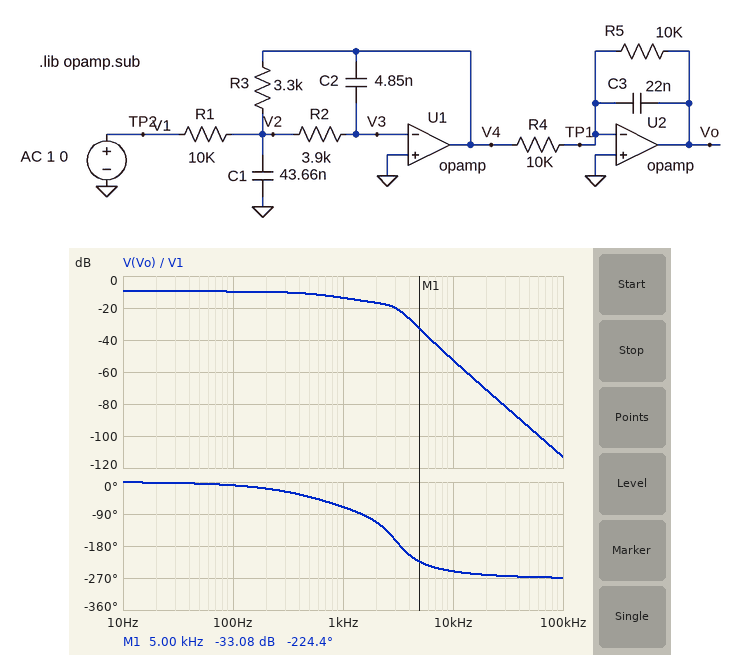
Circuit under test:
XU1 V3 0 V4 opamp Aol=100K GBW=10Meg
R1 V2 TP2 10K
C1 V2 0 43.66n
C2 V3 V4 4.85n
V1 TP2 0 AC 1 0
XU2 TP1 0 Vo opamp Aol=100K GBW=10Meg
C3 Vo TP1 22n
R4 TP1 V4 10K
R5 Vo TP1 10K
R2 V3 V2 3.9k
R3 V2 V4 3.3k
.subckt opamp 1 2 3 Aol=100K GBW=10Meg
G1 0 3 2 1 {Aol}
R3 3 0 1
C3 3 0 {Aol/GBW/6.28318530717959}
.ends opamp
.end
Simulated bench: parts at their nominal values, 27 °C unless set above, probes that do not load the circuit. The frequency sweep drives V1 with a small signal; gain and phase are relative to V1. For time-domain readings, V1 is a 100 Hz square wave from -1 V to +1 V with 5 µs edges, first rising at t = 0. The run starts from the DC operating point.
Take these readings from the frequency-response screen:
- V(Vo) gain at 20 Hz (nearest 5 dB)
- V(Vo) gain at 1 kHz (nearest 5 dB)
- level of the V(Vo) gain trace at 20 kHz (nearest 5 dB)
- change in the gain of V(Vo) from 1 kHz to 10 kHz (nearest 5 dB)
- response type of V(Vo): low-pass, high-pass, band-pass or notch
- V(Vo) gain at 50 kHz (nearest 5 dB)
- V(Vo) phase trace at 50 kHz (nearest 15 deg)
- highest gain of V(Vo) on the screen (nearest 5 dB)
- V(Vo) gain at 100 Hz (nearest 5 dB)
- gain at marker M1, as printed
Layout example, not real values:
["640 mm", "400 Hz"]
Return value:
["-10 dB", "-15 dB", "-70 dB", "-40 dB", "low-pass", "-95 dB", "-270 deg", "-10 dB", "-10 dB", "-33.08 dB"]
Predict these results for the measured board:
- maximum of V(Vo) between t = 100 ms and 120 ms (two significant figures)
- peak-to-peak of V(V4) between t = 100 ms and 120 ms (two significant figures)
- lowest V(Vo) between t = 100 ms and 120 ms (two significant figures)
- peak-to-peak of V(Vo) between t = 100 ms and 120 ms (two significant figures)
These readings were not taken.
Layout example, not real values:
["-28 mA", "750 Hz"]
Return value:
["330 mV", "1.0 V", "-330 mV", "660 mV"]
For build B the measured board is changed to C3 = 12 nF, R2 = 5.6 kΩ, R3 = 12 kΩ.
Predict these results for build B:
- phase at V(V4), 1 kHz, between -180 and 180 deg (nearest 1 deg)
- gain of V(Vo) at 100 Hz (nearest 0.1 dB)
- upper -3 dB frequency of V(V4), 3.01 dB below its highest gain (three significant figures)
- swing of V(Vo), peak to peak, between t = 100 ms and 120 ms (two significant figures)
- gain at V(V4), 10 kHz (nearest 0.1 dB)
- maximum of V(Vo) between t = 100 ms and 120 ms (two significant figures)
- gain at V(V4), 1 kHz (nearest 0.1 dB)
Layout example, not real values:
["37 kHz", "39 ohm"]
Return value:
["121 deg", "1.6 dB", "1.56 kHz", "2.8 V", "-33.3 dB", "1.4 V", "2.9 dB"]
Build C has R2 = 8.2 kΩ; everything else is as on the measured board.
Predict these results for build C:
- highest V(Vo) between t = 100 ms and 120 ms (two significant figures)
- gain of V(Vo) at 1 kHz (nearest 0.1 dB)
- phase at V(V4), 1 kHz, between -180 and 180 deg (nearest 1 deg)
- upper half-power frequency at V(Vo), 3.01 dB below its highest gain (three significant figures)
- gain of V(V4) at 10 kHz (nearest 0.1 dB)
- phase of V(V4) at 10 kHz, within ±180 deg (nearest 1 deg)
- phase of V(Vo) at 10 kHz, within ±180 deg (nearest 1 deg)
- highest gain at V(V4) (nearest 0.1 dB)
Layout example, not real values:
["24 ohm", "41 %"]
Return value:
["330 mV", "-13.2 dB", "151 deg", "856 Hz", "-36.5 dB", "11 deg", "105 deg", "-7.8 dB"]
